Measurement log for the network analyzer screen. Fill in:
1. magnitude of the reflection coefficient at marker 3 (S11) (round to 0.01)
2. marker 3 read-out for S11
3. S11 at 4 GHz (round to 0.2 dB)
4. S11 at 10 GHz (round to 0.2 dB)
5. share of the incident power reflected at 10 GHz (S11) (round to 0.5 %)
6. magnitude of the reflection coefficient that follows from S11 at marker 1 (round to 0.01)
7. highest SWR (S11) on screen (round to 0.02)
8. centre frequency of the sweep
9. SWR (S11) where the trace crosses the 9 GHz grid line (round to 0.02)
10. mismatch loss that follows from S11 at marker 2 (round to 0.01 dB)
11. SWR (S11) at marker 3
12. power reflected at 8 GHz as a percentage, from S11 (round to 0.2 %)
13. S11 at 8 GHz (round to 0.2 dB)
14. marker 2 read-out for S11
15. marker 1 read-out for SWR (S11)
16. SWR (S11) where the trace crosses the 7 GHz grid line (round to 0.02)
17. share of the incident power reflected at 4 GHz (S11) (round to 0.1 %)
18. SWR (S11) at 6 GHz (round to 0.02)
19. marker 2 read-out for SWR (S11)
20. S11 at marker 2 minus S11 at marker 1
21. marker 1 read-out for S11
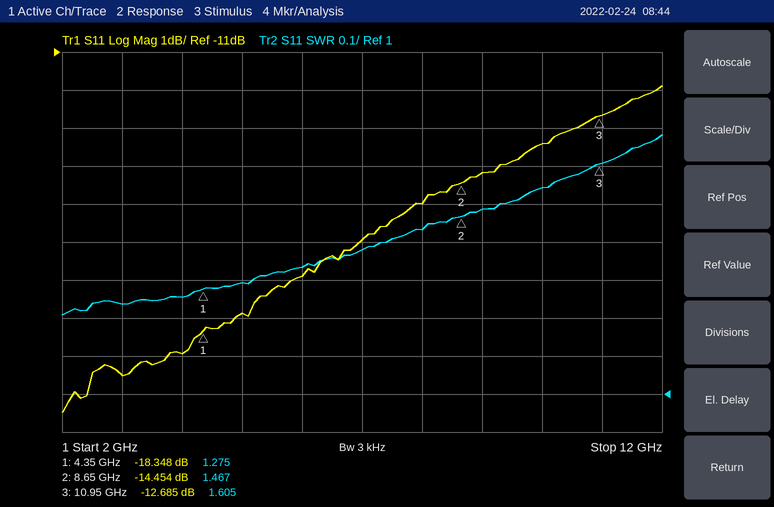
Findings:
0.23
-12.685 dB
-19.0 dB
-13.4 dB
4.5 %
0.12
1.68
7 GHz
1.48
0.16 dB
1.605
3.2 %
-15.0 dB
-14.454 dB
1.275
1.38
1.3 %
1.34
1.467
3.894 dB
-18.348 dB
